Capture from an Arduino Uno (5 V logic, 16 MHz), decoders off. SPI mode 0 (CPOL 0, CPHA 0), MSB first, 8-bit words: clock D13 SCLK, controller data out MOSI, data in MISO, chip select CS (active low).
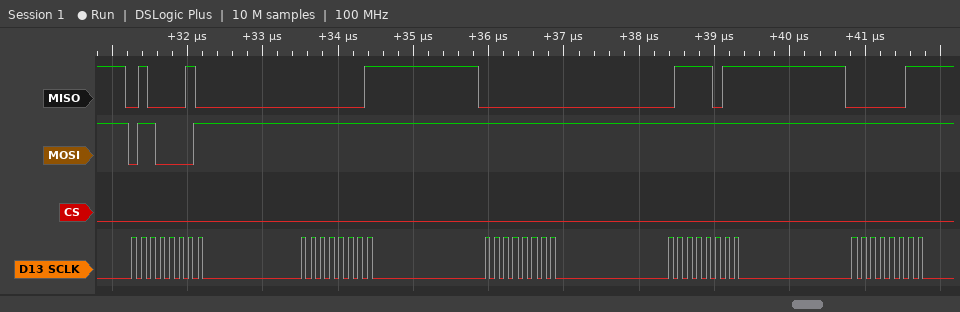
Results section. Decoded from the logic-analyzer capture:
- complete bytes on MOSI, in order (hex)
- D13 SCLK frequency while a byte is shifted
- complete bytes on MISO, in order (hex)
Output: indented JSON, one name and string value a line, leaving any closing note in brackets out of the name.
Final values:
{
  "complete bytes on MOSI, in order": "61 FF FF FF FF",
  "D13 SCLK frequency while a byte is shifted": "8 MHz",
  "complete bytes on MISO, in order": "42 01 00 7B 03"
}
